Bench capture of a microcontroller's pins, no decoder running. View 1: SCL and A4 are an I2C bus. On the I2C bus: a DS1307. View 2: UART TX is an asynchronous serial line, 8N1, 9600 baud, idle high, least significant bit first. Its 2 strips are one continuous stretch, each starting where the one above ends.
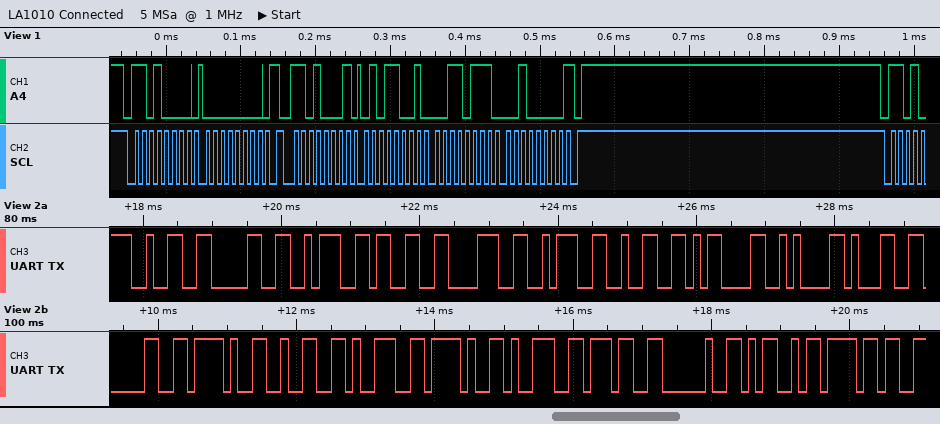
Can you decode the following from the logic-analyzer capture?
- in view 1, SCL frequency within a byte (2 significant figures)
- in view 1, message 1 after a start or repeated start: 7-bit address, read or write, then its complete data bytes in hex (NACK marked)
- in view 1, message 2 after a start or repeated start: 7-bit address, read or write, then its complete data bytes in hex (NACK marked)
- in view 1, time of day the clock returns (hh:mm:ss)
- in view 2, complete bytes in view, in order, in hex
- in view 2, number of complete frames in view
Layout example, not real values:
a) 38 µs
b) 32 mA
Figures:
a) 100 kHz
b) 0x68 write: 00
c) 0x68 read: 59 37 20 NACK
d) 20:37:59
e) 32 30 3A 33 38 3A 32 0D 0A 31 30 2F 32 39 2F 39 37 20 4D 6F
f) 20
